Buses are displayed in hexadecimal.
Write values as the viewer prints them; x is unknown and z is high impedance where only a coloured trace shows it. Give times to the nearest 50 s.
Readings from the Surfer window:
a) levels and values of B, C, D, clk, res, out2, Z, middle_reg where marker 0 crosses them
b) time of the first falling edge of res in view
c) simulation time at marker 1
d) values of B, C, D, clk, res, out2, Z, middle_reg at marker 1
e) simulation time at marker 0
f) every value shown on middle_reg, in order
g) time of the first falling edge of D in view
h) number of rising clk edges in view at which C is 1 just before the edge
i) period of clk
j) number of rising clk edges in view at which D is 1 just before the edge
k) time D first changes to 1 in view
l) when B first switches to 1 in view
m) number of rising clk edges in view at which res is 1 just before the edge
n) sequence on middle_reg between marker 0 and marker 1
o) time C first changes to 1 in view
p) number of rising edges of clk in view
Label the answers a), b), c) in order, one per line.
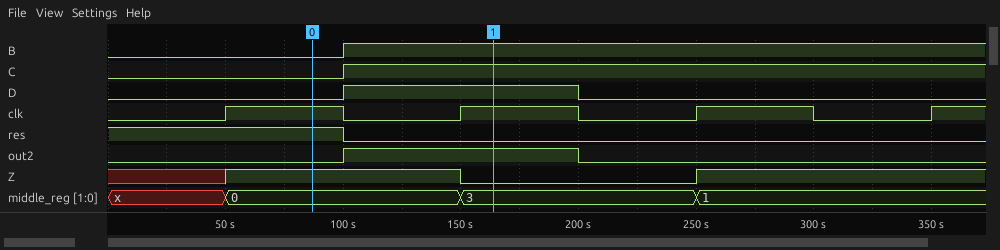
a) B=0, C=0, D=0, clk=1, res=1, out2=0, Z=1, middle_reg=0
b) 100 s
c) 150 s
d) B=1, C=1, D=1, clk=1, res=0, out2=1, Z=0, middle_reg=3
e) 100 s
f) x, 0, 3, 1
g) 200 s
h) 3
i) 100 s
j) 1
k) 100 s
l) 100 s
m) 1
n) 0, 3
o) 100 s
p) 4
